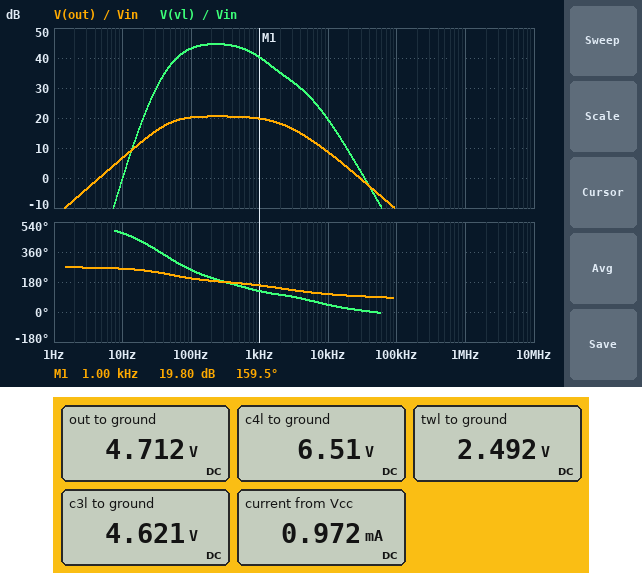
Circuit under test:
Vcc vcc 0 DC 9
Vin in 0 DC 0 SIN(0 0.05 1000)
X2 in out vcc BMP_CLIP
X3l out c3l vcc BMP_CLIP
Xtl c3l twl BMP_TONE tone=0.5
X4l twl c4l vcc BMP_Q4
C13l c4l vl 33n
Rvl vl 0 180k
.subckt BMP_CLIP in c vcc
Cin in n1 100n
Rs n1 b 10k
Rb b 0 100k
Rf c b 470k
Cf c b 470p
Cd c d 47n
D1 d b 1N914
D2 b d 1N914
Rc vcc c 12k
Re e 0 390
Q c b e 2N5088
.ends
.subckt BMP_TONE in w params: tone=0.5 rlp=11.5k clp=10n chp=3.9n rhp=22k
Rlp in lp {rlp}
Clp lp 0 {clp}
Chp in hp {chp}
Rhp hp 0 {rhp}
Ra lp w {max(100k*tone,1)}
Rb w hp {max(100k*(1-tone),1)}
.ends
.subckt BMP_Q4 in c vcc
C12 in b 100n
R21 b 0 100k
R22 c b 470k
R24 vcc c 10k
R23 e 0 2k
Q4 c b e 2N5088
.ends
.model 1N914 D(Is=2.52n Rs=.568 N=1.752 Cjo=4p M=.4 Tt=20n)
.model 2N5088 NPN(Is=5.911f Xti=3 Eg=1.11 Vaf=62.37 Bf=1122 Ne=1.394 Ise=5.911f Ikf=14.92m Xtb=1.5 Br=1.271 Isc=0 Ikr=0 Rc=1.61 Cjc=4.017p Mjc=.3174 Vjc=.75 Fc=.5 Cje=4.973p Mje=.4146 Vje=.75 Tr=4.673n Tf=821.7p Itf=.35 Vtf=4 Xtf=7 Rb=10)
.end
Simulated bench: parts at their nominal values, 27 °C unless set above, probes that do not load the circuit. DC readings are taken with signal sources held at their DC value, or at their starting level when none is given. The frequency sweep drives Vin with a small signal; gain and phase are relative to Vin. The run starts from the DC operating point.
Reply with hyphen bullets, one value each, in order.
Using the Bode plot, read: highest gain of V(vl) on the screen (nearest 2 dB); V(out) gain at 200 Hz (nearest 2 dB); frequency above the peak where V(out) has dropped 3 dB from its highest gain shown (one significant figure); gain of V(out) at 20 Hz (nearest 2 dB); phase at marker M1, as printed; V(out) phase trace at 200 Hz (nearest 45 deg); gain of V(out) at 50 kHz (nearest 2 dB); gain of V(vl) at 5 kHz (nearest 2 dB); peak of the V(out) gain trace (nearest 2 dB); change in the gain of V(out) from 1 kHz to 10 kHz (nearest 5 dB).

- 44 dB
- 20 dB
- 2 kHz
- 12 dB
- 159.5 deg
- 180 deg
- -4 dB
- 28 dB
- 20 dB
- -10 dB
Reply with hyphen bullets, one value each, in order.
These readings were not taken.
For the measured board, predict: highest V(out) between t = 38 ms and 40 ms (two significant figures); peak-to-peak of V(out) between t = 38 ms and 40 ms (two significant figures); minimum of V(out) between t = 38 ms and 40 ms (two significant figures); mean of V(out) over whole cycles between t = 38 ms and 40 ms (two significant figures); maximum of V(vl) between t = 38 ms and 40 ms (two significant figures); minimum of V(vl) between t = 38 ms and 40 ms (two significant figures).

- 5.0 V
- 540 mV
- 4.4 V
- 4.7 V
- 520 mV
- -530 mV
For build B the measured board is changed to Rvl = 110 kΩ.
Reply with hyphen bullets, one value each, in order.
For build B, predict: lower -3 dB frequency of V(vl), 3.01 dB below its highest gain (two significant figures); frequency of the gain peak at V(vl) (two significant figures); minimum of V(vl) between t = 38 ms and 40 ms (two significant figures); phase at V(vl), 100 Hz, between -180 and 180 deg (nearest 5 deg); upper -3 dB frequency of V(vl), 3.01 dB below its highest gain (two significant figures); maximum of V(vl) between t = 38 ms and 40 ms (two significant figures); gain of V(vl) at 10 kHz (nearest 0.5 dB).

- 81 Hz
- 240 Hz
- -510 mV
- -100 deg
- 800 Hz
- 500 mV
- 19.0 dB
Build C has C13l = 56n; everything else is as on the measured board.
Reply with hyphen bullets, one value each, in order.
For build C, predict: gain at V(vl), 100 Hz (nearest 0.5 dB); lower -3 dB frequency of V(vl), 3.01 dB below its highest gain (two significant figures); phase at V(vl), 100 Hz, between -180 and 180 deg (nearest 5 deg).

- 43.5 dB
- 72 Hz
- -115 deg
